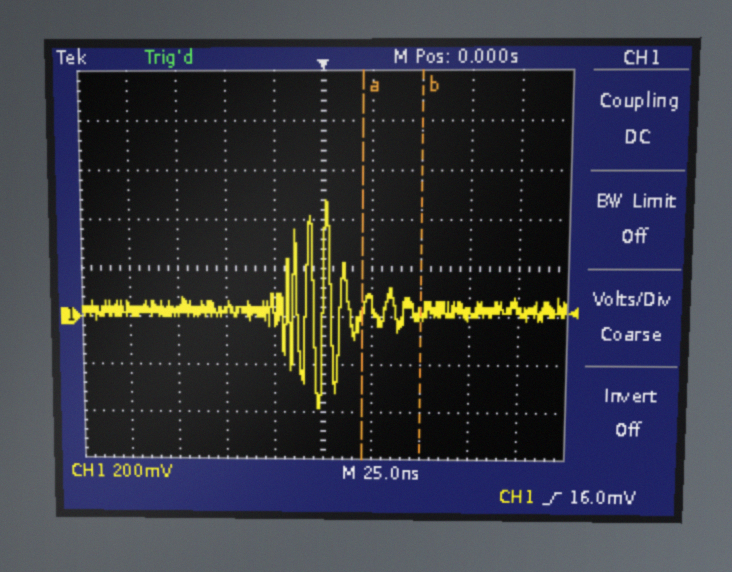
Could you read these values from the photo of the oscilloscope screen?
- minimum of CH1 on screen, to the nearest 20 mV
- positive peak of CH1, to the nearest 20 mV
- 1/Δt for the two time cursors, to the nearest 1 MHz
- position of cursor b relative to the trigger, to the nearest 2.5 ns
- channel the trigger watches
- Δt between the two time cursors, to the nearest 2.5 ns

-380 mV
480 mV
33 MHz
+50.0 ns
CH1
30.0 ns
